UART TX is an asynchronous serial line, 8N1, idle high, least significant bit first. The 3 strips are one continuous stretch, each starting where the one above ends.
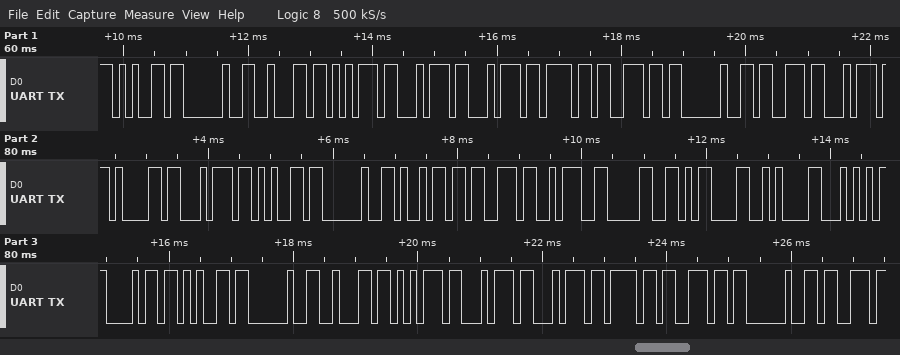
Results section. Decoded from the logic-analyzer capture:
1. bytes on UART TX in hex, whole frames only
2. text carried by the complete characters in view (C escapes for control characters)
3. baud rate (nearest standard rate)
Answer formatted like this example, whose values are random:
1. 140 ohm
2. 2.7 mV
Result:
1. 65 20 62 75 74 74 6F 6E 20 73 74 61 74 65 20 69 73 3A 30 0D 0A 54 68 65 20 62 75 74 74 6F 6E 20 73
2. "e button state is:0\r\nThe button s"
3. 9600 baud
